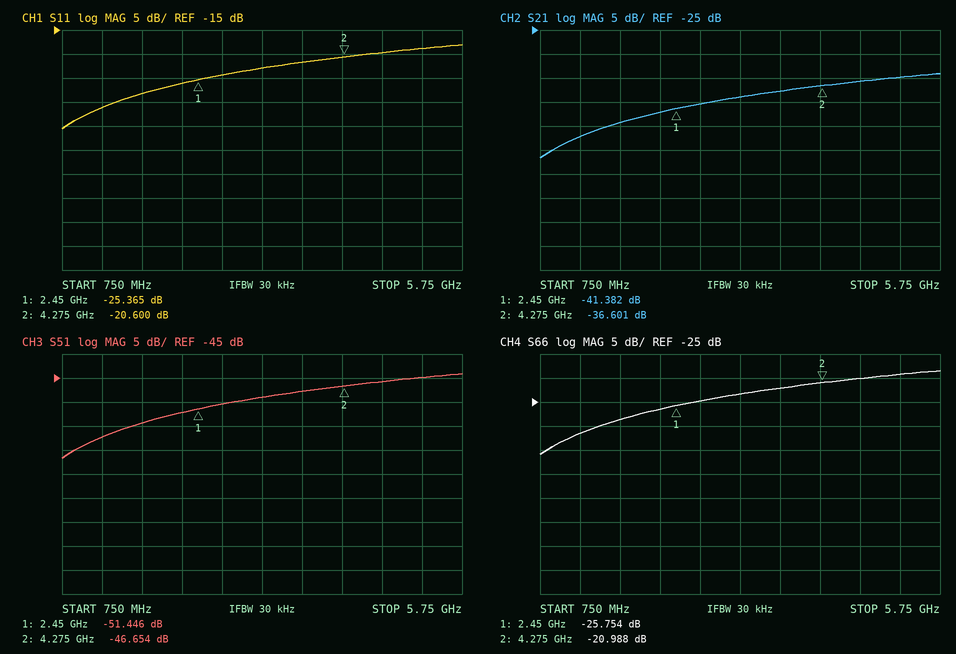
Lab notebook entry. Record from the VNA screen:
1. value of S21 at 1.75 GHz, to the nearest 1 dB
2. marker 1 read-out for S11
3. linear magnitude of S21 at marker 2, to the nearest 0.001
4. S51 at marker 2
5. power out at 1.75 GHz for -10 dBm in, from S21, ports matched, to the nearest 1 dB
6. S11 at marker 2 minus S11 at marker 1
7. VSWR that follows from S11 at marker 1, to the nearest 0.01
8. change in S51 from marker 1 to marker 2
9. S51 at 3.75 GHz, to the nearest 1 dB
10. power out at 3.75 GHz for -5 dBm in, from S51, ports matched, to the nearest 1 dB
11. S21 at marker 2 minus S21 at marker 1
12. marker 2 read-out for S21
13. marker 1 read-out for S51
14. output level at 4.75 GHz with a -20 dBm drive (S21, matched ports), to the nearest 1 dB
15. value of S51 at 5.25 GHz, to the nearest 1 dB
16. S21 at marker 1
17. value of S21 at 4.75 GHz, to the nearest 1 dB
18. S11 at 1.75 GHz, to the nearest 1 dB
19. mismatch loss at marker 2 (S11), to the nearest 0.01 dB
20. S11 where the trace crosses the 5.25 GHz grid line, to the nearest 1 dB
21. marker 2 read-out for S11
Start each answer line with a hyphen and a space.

- -44 dB
- -25.365 dB
- 0.015
- -46.654 dB
- -54 dBm
- 4.765 dB
- 1.11
- 4.792 dB
- -48 dB
- -53 dBm
- 4.781 dB
- -36.601 dB
- -51.446 dB
- -56 dBm
- -45 dB
- -41.382 dB
- -36 dB
- -28 dB
- 0.04 dB
- -19 dB
- -20.600 dB
